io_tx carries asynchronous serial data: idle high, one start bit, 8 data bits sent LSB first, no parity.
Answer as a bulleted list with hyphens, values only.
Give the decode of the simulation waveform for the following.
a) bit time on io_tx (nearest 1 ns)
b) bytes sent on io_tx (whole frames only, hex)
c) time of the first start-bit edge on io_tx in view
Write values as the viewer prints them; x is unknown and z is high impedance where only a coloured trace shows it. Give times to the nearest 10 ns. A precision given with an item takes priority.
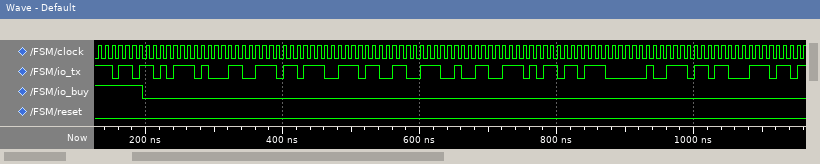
- 10 ns
- 5B, 31, 3B, 33, 32, 6D, 20, 1B
- 150 ns
